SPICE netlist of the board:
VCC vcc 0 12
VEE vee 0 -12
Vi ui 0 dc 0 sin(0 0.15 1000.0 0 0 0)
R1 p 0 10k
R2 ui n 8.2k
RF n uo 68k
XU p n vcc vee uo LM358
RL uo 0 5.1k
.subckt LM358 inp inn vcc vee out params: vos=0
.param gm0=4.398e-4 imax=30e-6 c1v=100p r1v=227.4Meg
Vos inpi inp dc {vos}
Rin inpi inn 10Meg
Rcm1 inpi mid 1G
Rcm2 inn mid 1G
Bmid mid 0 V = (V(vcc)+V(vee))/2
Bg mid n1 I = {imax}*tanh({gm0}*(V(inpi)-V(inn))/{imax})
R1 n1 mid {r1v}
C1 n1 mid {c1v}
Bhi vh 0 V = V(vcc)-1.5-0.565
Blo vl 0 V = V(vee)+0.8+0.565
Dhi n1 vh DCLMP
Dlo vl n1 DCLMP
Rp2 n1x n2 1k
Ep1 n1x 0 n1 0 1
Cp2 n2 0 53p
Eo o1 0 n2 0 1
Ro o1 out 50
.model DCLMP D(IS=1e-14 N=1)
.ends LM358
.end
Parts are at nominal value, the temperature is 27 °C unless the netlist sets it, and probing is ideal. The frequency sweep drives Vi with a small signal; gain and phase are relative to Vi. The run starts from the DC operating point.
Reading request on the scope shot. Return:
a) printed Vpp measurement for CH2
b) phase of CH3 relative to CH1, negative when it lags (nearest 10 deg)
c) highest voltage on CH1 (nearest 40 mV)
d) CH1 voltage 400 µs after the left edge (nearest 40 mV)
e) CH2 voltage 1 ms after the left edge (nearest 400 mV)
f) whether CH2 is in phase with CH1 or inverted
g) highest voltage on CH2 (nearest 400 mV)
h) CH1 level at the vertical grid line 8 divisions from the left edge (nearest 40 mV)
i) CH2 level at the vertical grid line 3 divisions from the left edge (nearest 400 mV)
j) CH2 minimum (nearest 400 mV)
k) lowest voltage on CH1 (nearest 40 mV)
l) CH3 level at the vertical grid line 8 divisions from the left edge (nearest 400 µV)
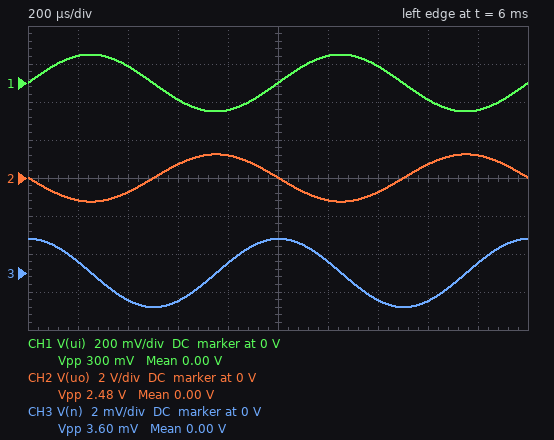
2.48 V
90 deg
160 mV
80 mV
0 V
inverted
1.2 V
-80 mV
800 mV
-1.2 V
-160 mV
-1.6 mV
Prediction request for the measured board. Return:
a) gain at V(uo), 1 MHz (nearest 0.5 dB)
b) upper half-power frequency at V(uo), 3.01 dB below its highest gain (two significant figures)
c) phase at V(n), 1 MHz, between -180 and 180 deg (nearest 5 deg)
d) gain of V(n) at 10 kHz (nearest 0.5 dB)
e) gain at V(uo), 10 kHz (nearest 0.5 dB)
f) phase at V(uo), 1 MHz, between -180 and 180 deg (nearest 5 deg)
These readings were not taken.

-4.5 dB
76 kHz
5 deg
-18.5 dB
18.5 dB
75 deg
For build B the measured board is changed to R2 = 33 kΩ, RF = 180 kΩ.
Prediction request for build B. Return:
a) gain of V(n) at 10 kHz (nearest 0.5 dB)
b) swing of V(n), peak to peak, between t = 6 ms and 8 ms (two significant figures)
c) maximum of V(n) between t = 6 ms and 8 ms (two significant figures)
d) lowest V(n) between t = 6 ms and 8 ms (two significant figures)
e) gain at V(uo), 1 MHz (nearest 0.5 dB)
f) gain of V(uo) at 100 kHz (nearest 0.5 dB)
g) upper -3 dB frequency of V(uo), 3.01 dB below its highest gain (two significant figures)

-22.0 dB
2.4 mV
1.2 mV
-1.2 mV
-5.0 dB
12.0 dB
110 kHz
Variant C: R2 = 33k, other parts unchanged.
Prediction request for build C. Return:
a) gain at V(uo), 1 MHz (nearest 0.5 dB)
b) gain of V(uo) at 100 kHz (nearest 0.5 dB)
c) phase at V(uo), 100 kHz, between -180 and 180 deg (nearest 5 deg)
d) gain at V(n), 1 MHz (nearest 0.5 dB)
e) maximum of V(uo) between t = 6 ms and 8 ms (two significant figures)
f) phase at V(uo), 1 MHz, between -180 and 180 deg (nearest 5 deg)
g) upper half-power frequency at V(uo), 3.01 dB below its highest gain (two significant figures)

-6.5 dB
5.5 dB
155 deg
-3.0 dB
310 mV
85 deg
240 kHz
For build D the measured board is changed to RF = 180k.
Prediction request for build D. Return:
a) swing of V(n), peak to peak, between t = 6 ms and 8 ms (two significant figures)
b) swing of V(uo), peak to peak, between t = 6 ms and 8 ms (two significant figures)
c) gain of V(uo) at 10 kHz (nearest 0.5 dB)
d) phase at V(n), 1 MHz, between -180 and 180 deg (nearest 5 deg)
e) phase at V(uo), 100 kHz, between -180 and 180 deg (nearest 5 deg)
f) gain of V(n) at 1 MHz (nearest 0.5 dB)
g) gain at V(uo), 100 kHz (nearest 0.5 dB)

9.5 mV
6.6 V
26.5 dB
0 deg
105 deg
-0.5 dB
16.0 dB
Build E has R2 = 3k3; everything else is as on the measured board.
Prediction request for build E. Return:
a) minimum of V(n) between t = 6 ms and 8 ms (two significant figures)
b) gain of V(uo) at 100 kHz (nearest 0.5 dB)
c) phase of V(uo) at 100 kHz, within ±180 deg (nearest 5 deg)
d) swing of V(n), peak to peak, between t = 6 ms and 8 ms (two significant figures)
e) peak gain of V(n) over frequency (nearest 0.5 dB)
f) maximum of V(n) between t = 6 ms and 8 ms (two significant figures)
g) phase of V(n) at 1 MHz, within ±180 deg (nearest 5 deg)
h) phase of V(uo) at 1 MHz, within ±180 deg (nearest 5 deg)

-4.5 mV
16.0 dB
105 deg
8.9 mV
-0.5 dB
4.5 mV
0 deg
75 deg
